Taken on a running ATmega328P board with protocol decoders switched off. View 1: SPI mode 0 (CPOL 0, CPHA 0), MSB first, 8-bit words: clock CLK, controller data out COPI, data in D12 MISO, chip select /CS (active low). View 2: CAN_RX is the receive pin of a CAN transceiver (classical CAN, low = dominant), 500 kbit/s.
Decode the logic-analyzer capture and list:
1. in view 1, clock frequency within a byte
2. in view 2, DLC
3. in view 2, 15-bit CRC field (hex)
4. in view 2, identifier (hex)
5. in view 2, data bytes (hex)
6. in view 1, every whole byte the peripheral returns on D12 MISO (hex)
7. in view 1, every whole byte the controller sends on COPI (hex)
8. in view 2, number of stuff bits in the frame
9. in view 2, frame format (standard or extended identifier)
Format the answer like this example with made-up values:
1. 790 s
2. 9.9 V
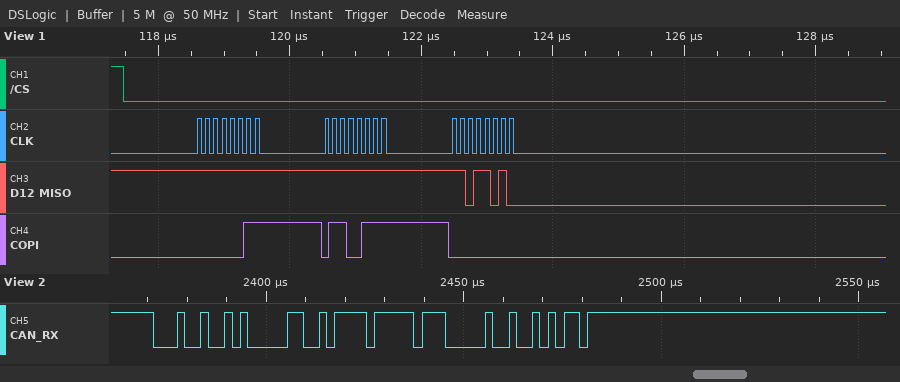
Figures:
1. 8 MHz
2. 2
3. 0x0095
4. 0x125
5. 5E FF
6. FF FF DA
7. 03 67 00
8. 3
9. standard
